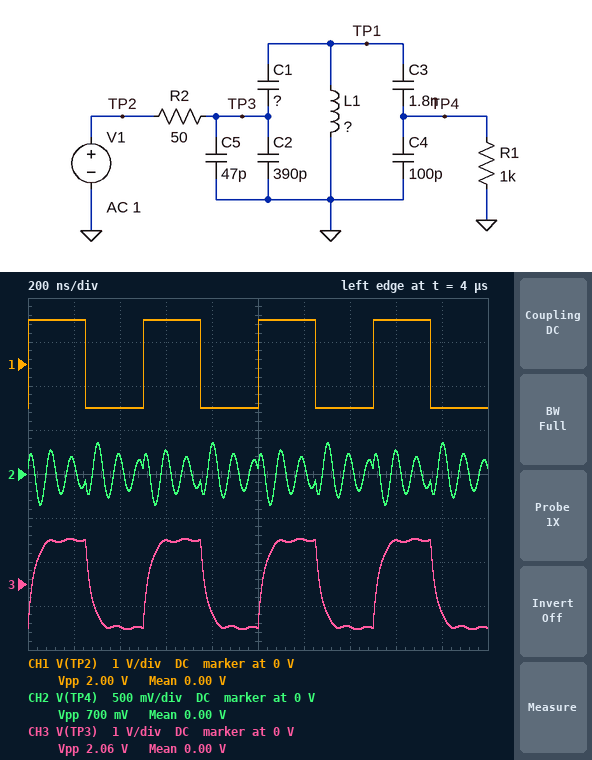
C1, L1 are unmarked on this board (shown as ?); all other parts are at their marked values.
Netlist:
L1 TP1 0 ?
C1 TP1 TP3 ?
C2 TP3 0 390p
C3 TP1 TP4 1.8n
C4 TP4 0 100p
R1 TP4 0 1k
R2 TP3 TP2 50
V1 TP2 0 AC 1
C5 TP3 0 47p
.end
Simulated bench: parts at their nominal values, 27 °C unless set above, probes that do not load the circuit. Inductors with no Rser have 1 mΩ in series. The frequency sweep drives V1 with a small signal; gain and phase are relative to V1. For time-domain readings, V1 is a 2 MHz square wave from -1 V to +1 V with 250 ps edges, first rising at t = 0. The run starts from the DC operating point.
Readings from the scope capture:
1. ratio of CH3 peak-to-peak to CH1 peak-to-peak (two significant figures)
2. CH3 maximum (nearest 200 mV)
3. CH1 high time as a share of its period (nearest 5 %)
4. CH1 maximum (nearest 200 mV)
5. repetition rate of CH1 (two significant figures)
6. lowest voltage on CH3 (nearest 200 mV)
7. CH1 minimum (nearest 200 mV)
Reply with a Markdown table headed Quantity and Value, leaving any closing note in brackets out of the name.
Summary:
| Quantity | Value |
|---|---|
| ratio of CH3 peak-to-peak to CH1 peak-to-peak | 1.0 |
| CH3 maximum | 1.0 V |
| CH1 high time as a share of its period | 50 % |
| CH1 maximum | 1.0 V |
| repetition rate of CH1 | 2.0 MHz |
| lowest voltage on CH3 | -1.0 V |
| CH1 minimum | -1.0 V |
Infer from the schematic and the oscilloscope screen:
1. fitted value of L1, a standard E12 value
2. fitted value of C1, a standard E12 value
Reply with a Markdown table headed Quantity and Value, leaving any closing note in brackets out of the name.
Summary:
| Quantity | Value |
|---|---|
| fitted value of L1, a standard E12 value | 1.2 µH |
| fitted value of C1, a standard E12 value | 82 pF |
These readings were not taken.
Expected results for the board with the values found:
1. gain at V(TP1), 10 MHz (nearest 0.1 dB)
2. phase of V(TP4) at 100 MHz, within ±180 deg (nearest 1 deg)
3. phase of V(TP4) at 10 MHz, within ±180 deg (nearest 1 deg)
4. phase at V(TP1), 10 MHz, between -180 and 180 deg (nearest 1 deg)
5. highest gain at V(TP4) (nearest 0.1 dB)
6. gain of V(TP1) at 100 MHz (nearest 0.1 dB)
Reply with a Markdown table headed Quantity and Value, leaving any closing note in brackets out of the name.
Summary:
| Quantity | Value |
|---|---|
| gain at V(TP1), 10 MHz | -1.0 dB |
| phase of V(TP4) at 100 MHz, within ±180 deg | -86 deg |
| phase of V(TP4) at 10 MHz, within ±180 deg | 97 deg |
| phase at V(TP1), 10 MHz, between -180 and 180 deg | 97 deg |
| highest gain at V(TP4) | 6.2 dB |
| gain of V(TP1) at 100 MHz | -30.2 dB |
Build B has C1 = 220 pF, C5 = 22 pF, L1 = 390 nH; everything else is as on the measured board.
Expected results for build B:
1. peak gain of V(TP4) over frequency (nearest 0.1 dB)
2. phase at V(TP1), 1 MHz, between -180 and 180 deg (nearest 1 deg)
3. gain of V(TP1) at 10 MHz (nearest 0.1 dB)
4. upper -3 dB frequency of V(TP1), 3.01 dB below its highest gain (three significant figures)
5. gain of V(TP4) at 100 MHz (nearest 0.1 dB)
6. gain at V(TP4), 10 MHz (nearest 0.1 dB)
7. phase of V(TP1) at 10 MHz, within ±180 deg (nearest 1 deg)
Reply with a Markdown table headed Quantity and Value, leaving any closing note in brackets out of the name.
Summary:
| Quantity | Value |
|---|---|
| peak gain of V(TP4) over frequency | 6.1 dB |
| phase at V(TP1), 1 MHz, between -180 and 180 deg | 169 deg |
| gain of V(TP1) at 10 MHz | -12.1 dB |
| upper -3 dB frequency of V(TP1), 3.01 dB below its highest gain | 17.4 MHz |
| gain of V(TP4) at 100 MHz | -26.9 dB |
| gain at V(TP4), 10 MHz | -12.6 dB |
| phase of V(TP1) at 10 MHz, within ±180 deg | 110 deg |
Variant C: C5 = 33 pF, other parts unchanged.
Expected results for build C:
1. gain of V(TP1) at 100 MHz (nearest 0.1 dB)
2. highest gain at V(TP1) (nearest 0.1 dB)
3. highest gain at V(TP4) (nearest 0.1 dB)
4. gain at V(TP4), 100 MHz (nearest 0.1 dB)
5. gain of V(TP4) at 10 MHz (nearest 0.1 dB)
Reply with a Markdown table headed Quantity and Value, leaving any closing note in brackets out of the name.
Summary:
| Quantity | Value |
|---|---|
| gain of V(TP1) at 100 MHz | -29.9 dB |
| highest gain at V(TP1) | 6.8 dB |
| highest gain at V(TP4) | 6.3 dB |
| gain at V(TP4), 100 MHz | -30.4 dB |
| gain of V(TP4) at 10 MHz | -1.3 dB |
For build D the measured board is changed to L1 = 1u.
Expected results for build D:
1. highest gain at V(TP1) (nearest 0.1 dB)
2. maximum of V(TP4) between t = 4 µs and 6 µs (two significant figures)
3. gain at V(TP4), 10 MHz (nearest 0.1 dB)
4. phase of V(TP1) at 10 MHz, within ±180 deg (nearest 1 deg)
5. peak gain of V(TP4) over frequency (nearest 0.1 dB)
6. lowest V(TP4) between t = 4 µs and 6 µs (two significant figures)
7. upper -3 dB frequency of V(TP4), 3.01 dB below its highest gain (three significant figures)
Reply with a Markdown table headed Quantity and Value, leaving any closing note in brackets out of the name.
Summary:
| Quantity | Value |
|---|---|
| highest gain at V(TP1) | 6.8 dB |
| maximum of V(TP4) between t = 4 µs and 6 µs | 280 mV |
| gain at V(TP4), 10 MHz | -6.7 dB |
| phase of V(TP1) at 10 MHz, within ±180 deg | 108 deg |
| peak gain of V(TP4) over frequency | 6.3 dB |
| lowest V(TP4) between t = 4 µs and 6 µs | -280 mV |
| upper -3 dB frequency of V(TP4), 3.01 dB below its highest gain | 13.0 MHz |
